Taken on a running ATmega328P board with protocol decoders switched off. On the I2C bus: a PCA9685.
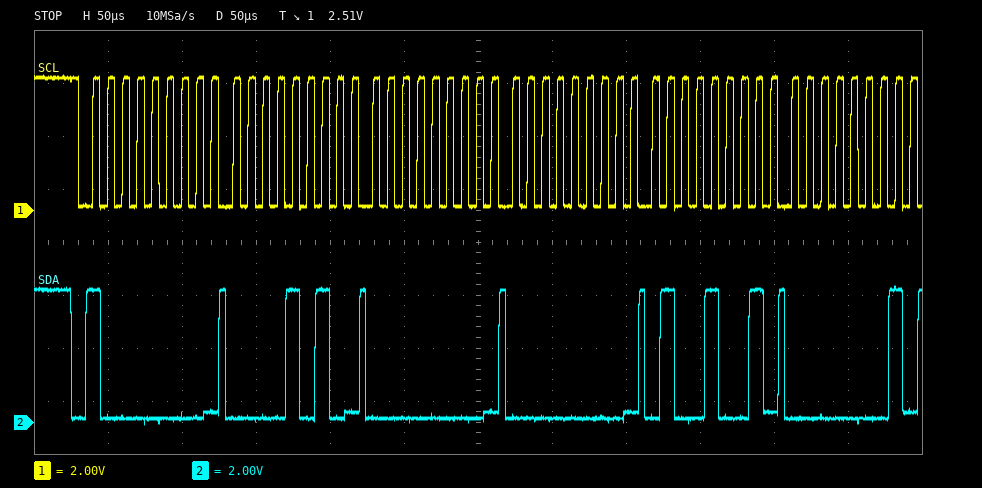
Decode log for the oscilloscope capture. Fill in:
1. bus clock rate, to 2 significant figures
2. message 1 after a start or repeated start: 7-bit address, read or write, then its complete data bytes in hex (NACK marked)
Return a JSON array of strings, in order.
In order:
["100 kHz", "0x40 write: 0A 00 00 49 01"]
